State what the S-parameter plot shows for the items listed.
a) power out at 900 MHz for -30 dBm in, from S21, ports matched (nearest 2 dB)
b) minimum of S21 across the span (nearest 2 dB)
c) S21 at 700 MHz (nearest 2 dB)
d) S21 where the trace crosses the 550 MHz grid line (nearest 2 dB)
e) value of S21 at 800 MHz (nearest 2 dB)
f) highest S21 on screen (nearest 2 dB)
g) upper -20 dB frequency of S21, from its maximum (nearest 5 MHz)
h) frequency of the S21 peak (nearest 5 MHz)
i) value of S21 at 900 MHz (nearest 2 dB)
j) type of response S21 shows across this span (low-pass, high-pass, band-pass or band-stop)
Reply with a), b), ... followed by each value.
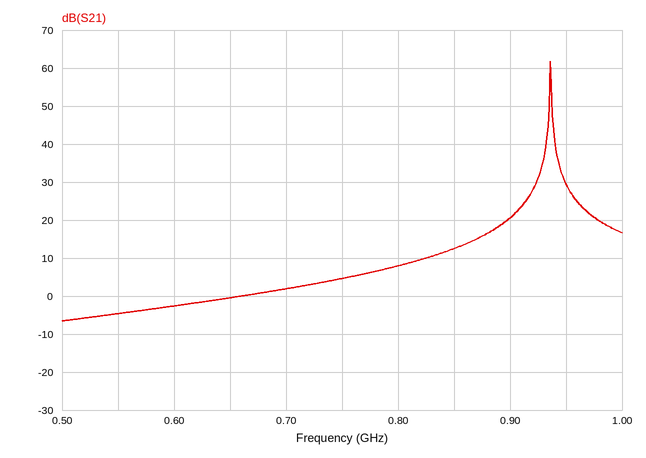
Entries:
a) -10 dBm
b) -6 dB
c) 2 dB
d) -4 dB
e) 8 dB
f) 62 dB
g) 940 MHz
h) 935 MHz
i) 20 dB
j) band-pass
